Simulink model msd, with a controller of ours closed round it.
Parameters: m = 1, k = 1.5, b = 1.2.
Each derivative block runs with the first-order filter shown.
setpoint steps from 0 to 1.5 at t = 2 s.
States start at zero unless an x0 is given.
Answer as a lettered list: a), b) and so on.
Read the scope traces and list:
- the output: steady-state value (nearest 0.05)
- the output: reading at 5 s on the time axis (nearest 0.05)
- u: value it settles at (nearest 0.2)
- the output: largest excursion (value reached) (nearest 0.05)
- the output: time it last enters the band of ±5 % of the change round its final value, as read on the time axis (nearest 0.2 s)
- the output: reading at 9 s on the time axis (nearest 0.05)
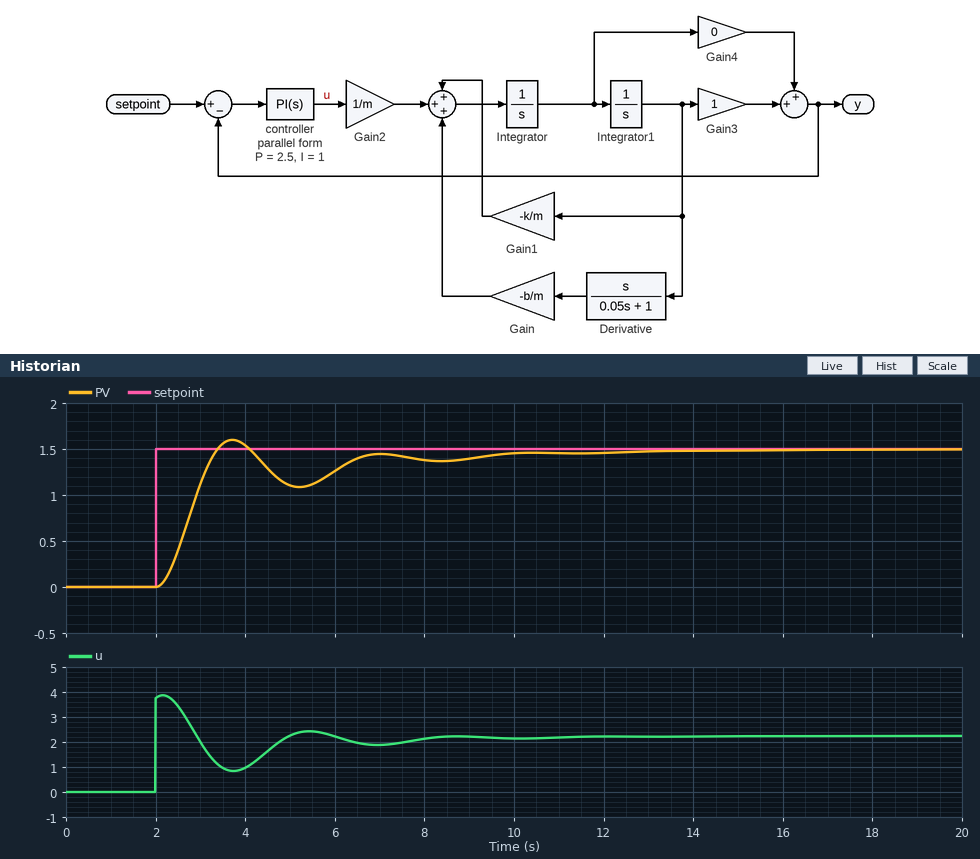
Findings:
a) 1.50
b) 1.10
c) 2.2
d) 1.60
e) 9.4 s
f) 1.40
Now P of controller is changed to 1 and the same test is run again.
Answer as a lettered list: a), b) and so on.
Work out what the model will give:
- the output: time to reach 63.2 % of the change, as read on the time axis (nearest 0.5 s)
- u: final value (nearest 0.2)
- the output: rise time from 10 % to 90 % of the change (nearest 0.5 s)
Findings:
a) 3.5 s
b) 2.2
c) 1.5 s
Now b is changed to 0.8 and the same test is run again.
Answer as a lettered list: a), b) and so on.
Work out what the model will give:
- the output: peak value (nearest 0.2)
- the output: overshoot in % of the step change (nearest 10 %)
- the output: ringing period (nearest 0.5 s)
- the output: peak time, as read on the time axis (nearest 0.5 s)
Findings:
a) 1.8
b) 20 %
c) 3.0 s
d) 3.5 s
